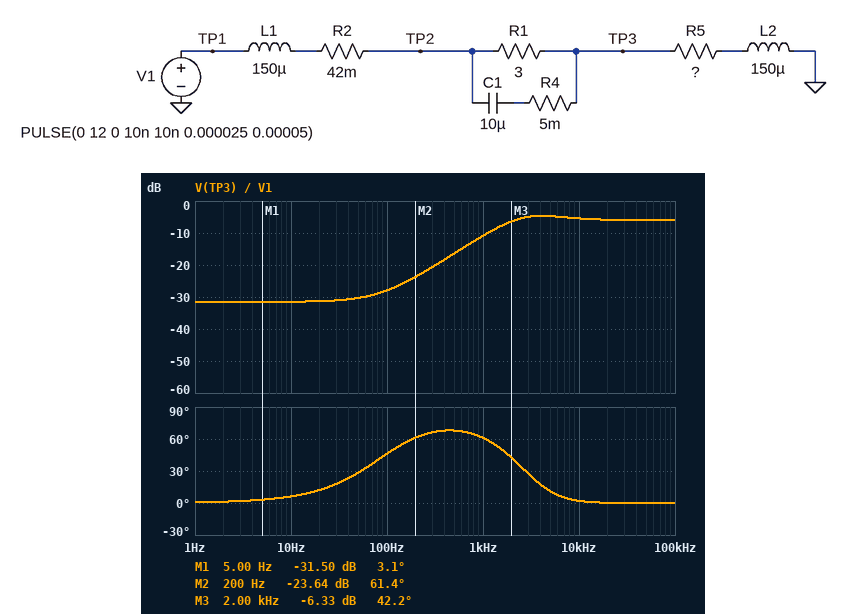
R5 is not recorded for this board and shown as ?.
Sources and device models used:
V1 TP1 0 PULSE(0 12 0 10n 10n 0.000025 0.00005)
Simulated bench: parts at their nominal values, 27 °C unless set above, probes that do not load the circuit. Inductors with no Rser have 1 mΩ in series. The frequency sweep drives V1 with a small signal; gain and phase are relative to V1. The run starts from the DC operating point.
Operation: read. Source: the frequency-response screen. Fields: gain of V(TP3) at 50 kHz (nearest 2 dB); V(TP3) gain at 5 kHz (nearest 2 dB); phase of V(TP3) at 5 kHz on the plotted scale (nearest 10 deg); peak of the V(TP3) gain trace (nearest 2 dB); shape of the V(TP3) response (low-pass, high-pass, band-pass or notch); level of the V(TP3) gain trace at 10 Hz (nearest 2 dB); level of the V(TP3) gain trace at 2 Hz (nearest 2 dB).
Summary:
-6 dB
-4 dB
10 deg
-4 dB
high-pass
-32 dB
-32 dB
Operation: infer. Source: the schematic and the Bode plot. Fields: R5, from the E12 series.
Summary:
0.082 Ω
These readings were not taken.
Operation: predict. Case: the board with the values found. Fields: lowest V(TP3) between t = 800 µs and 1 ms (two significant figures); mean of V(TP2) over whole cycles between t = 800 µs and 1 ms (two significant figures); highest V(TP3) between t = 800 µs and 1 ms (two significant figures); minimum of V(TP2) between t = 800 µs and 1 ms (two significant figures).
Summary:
-2.9 V
5.9 V
3.2 V
2.9 V
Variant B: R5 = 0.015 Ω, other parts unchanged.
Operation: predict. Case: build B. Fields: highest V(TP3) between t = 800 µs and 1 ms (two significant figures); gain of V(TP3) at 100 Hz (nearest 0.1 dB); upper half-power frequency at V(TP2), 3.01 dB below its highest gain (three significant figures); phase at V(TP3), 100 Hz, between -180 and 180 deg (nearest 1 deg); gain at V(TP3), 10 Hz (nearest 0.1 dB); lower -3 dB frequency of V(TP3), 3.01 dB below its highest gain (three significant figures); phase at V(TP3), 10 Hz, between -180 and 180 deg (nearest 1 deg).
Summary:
3.1 V
-30.1 dB
2.13 kHz
78 deg
-44.3 dB
1.56 kHz
30 deg
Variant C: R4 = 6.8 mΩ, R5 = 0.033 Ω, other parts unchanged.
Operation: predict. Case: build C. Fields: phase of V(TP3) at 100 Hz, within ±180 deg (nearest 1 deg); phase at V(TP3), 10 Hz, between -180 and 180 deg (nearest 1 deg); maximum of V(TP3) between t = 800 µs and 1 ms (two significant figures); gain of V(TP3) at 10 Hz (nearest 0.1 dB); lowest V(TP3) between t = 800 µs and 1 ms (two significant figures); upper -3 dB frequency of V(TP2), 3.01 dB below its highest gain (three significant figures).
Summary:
68 deg
15 deg
3.1 V
-38.8 dB
-3.0 V
2.14 kHz
